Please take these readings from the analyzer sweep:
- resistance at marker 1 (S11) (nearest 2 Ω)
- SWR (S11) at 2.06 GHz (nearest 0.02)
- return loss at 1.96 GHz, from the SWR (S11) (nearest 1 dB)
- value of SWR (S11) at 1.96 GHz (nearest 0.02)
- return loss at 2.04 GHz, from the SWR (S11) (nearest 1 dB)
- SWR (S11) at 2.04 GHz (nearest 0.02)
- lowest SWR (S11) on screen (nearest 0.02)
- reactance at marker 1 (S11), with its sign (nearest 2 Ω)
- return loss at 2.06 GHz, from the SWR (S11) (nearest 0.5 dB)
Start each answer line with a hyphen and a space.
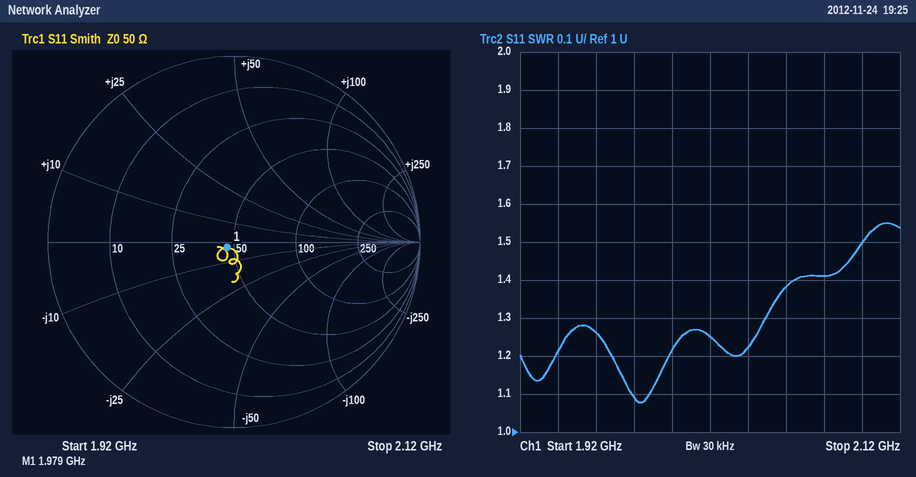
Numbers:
- 46 Ω
- 1.38
- 19 dB
- 1.26
- 20 dB
- 1.22
- 1.08
- -2 Ω
- 16.0 dB
